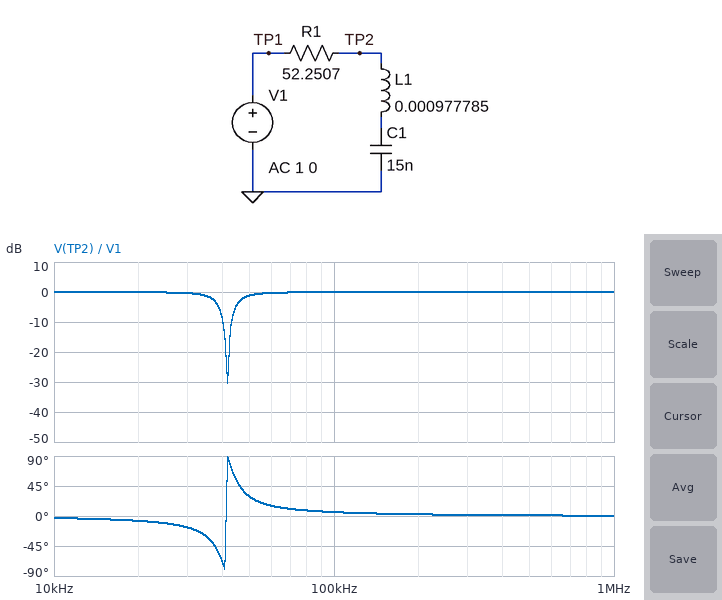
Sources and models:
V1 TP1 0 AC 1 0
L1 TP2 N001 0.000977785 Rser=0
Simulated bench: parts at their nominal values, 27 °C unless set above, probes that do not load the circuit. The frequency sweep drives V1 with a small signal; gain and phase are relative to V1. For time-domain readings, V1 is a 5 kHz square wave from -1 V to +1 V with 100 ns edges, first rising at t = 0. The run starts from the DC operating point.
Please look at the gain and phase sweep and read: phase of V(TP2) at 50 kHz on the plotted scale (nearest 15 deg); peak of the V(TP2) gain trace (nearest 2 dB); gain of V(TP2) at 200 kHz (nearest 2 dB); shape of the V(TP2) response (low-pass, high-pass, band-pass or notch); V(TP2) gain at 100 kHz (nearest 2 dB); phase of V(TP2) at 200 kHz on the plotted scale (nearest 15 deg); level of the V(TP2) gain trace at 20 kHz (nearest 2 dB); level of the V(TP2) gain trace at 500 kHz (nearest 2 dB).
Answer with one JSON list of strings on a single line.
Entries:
["30 deg", "0 dB", "0 dB", "notch", "0 dB", "0 deg", "0 dB", "0 dB"]
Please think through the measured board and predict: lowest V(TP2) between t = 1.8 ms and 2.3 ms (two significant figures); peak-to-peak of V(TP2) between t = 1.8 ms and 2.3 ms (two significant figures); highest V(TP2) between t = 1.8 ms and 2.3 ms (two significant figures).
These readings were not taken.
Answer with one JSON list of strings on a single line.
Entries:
["-1.2 V", "2.5 V", "1.2 V"]
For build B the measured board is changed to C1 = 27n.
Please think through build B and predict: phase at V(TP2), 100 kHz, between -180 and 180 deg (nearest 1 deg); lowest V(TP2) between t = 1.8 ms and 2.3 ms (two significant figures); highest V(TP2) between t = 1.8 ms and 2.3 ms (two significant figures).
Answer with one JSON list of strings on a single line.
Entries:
["5 deg", "-1.3 V", "1.3 V"]
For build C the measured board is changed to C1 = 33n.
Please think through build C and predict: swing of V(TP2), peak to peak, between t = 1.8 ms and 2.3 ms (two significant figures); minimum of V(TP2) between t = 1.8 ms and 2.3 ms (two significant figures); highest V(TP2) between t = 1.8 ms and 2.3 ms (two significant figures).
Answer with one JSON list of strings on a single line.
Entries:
["2.6 V", "-1.3 V", "1.3 V"]
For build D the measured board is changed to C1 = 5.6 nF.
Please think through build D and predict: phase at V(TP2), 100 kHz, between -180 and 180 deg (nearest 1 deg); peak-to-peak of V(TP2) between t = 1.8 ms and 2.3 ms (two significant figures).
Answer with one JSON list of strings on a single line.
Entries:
["9 deg", "2.4 V"]
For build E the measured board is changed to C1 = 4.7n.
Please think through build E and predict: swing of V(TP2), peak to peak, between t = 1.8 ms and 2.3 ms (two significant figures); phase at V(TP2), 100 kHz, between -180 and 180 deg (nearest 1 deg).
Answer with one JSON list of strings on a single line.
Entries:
["2.4 V", "11 deg"]
